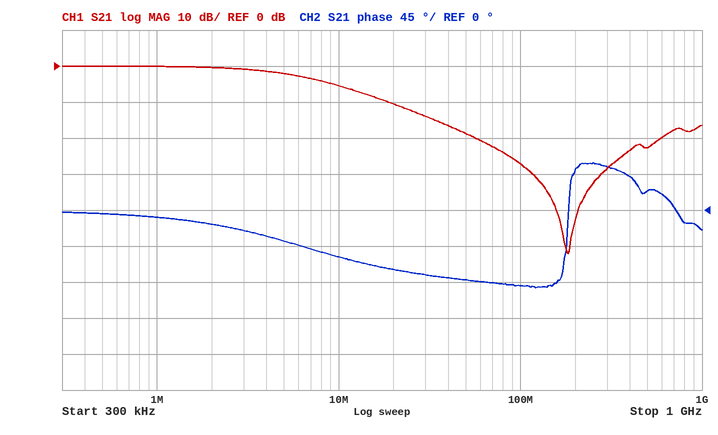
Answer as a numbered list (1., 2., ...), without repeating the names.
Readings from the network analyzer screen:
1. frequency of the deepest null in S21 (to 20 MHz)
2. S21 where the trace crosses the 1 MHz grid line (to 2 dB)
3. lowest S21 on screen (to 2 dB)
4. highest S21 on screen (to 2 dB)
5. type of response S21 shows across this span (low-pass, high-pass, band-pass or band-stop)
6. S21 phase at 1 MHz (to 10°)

1. 180 MHz
2. 0 dB
3. -52 dB
4. 0 dB
5. low-pass
6. -10°
